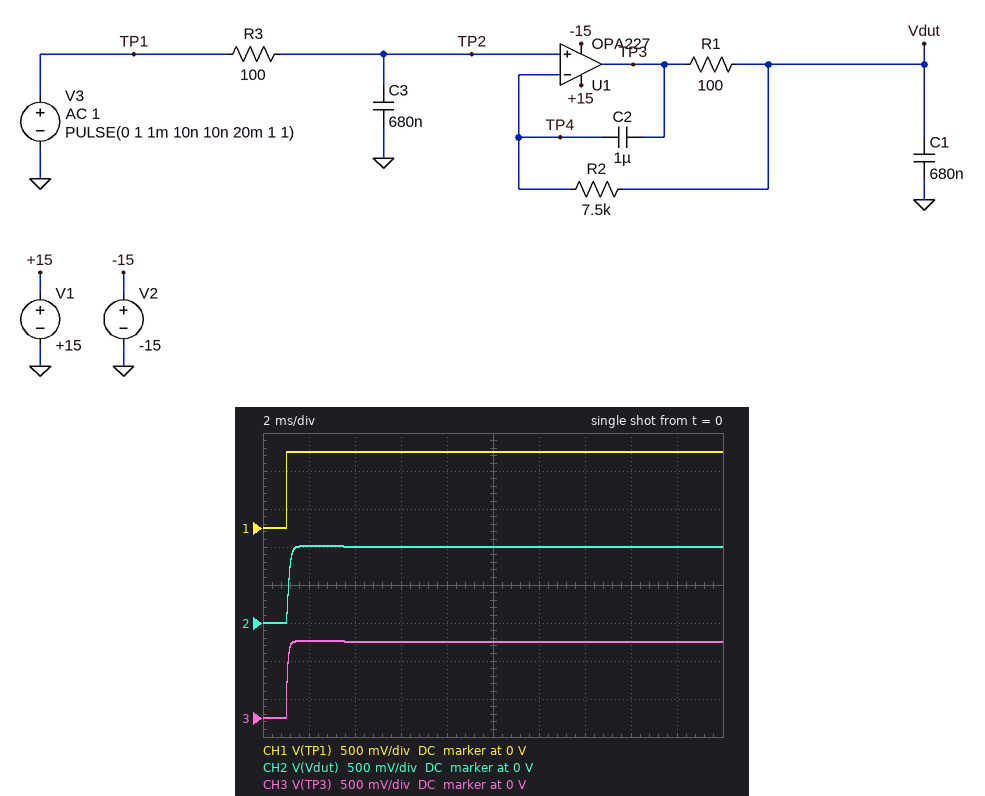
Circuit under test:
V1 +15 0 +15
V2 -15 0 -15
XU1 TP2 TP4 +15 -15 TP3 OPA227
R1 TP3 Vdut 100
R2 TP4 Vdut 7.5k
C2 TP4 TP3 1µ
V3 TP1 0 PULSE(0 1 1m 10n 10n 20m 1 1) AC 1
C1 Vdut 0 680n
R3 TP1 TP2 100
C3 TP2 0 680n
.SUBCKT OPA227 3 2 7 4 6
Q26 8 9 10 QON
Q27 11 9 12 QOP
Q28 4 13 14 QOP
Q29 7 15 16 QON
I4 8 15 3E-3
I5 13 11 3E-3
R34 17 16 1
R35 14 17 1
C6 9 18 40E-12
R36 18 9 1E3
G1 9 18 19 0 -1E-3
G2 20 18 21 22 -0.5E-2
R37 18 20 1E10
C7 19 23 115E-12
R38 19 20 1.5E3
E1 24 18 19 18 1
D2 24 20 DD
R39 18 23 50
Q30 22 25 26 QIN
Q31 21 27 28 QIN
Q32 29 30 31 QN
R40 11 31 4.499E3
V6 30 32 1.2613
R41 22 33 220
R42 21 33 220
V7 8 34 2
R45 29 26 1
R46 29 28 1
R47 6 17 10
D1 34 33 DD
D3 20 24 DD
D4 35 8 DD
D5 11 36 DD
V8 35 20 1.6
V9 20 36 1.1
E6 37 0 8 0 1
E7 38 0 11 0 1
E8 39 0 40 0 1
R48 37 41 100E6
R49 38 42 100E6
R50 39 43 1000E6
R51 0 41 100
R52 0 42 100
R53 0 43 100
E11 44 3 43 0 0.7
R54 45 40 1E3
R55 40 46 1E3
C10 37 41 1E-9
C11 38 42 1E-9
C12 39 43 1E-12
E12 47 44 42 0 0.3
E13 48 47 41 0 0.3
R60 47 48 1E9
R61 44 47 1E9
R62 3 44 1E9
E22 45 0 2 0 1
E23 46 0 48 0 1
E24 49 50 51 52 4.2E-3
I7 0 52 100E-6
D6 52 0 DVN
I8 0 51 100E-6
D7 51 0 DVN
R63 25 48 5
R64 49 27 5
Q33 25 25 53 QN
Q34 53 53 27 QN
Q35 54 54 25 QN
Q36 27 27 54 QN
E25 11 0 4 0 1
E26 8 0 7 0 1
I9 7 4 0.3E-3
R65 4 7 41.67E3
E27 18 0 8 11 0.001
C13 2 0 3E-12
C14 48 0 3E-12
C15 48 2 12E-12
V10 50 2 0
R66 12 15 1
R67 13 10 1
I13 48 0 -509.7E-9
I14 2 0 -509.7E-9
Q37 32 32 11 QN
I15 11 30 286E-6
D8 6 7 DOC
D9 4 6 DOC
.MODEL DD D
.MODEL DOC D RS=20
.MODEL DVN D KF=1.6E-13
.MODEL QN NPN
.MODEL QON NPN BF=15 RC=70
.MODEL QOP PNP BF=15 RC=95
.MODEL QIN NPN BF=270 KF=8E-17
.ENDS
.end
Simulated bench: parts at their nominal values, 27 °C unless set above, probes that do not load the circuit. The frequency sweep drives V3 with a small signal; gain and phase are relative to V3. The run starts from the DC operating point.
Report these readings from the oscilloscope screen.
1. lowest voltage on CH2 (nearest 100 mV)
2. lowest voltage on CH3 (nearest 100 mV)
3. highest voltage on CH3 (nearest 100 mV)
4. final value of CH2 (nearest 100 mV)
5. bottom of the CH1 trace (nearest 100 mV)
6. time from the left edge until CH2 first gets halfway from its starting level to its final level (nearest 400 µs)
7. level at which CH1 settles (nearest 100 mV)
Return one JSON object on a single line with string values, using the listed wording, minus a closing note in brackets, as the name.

{"lowest voltage on CH2": "0 V", "lowest voltage on CH3": "0 V", "highest voltage on CH3": "1.0 V", "final value of CH2": "1.0 V", "bottom of the CH1 trace": "0 V", "time from the left edge until CH2 first gets halfway from its starting level to its final level": "1.2 ms", "level at which CH1 settles": "1.0 V"}
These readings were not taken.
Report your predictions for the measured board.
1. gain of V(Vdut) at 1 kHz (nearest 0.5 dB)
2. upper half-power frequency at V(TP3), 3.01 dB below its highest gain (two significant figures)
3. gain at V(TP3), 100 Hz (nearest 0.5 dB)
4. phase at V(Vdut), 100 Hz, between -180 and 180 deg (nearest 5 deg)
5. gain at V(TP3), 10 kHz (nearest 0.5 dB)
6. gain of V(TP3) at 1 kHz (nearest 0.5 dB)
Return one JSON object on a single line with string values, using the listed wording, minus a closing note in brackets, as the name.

{"gain of V(Vdut) at 1 kHz": "-1.5 dB", "upper half-power frequency at V(TP3), 3.01 dB below its highest gain": "2.3 kHz", "gain at V(TP3), 100 Hz": "0 dB", "phase at V(Vdut), 100 Hz, between -180 and 180 deg": "-5 deg", "gain at V(TP3), 10 kHz": "-13.0 dB", "gain of V(TP3) at 1 kHz": "-0.5 dB"}
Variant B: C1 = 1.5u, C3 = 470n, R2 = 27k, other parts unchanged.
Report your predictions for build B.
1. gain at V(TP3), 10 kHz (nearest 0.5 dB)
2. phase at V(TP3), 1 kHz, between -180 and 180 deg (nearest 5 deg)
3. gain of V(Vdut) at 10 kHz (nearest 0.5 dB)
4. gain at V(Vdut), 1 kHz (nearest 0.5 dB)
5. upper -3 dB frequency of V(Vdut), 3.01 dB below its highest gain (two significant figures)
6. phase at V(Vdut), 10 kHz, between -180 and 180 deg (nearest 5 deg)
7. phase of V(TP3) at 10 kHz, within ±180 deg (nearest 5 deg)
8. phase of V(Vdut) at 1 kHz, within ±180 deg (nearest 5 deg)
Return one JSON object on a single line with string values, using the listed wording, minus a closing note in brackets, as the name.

{"gain at V(TP3), 10 kHz": "-10.0 dB", "phase at V(TP3), 1 kHz, between -180 and 180 deg": "-15 deg", "gain of V(Vdut) at 10 kHz": "-29.5 dB", "gain at V(Vdut), 1 kHz": "-3.0 dB", "upper -3 dB frequency of V(Vdut), 3.01 dB below its highest gain": "980 Hz", "phase at V(Vdut), 10 kHz, between -180 and 180 deg": "-155 deg", "phase of V(TP3) at 10 kHz, within ±180 deg": "-70 deg", "phase of V(Vdut) at 1 kHz, within ±180 deg": "-60 deg"}
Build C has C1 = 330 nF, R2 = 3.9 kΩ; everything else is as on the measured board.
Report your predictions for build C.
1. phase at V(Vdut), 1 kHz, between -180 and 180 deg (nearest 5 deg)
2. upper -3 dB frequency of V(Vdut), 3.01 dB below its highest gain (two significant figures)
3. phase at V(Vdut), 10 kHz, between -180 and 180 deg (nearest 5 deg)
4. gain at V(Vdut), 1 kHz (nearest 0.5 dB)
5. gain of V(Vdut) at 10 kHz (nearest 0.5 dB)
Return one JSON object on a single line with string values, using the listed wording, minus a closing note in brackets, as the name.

{"phase at V(Vdut), 1 kHz, between -180 and 180 deg": "-35 deg", "upper -3 dB frequency of V(Vdut), 3.01 dB below its highest gain": "2.0 kHz", "phase at V(Vdut), 10 kHz, between -180 and 180 deg": "-140 deg", "gain at V(Vdut), 1 kHz": "-1.0 dB", "gain of V(Vdut) at 10 kHz": "-20.0 dB"}
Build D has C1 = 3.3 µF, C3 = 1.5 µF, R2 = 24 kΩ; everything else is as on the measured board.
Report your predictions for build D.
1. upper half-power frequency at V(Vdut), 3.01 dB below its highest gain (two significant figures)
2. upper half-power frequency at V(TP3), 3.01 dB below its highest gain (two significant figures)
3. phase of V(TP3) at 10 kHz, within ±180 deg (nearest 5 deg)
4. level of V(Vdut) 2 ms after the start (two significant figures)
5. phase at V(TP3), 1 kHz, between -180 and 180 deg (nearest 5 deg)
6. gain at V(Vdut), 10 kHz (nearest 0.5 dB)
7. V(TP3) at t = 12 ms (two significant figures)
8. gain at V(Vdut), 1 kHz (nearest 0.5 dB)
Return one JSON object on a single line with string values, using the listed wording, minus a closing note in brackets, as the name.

{"upper half-power frequency at V(Vdut), 3.01 dB below its highest gain": "410 Hz", "upper half-power frequency at V(TP3), 3.01 dB below its highest gain": "1.0 kHz", "phase of V(TP3) at 10 kHz, within ±180 deg": "-85 deg", "level of V(Vdut) 2 ms after the start": "920 mV", "phase at V(TP3), 1 kHz, between -180 and 180 deg": "-45 deg", "gain at V(Vdut), 10 kHz": "-46.0 dB", "V(TP3) at t = 12 ms": "1.0 V", "gain at V(Vdut), 1 kHz": "-10.0 dB"}
